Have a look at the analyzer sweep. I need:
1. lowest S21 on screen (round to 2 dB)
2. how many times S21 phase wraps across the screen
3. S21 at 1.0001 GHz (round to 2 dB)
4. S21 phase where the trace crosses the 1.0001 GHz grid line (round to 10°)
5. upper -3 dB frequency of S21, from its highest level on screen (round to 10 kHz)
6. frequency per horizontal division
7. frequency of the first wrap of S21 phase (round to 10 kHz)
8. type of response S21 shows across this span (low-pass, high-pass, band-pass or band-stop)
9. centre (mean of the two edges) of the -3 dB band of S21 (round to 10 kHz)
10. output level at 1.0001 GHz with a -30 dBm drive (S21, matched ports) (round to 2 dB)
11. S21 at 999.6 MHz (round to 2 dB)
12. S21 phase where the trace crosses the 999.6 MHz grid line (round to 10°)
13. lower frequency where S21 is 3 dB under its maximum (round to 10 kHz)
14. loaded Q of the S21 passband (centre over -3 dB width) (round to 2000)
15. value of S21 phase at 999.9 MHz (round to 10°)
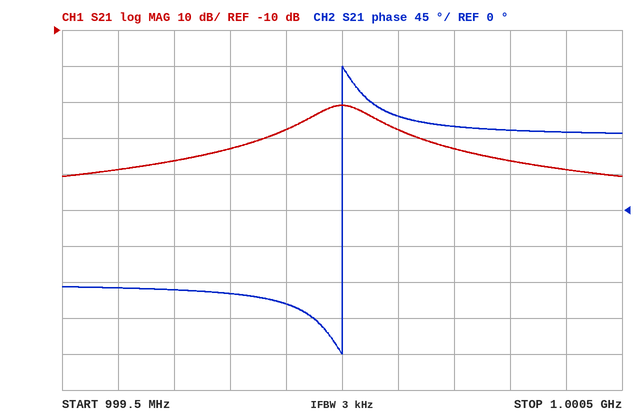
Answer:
-50 dB
1
-38 dB
120°
1.00005 GHz
100 kHz
1.00000 GHz
band-pass
1.00000 GHz
-68 dBm
-48 dB
-100°
999.95 MHz
10000
-120°
